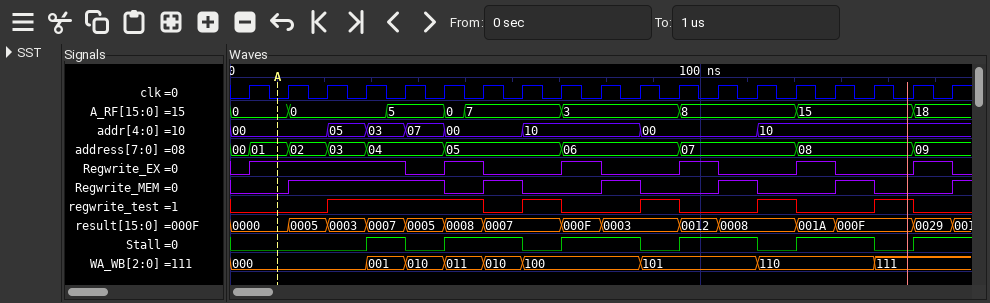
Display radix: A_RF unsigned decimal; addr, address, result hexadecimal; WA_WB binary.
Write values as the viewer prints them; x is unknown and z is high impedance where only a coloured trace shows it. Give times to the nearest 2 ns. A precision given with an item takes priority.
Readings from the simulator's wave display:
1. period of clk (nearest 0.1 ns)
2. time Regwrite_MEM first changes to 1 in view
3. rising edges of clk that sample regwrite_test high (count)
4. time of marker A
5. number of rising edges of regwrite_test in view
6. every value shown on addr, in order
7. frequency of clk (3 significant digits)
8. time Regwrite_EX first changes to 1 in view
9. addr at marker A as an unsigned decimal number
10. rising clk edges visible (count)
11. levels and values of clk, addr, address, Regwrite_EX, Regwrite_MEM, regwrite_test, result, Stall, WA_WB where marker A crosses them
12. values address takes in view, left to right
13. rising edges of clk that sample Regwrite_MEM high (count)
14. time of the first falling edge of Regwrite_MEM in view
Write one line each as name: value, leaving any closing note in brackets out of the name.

period of clk: 8.3 ns
time Regwrite_MEM first changes to 1 in view: 12 ns
rising edges of clk that sample regwrite_test high: 8
time of marker A: 10 ns
number of rising edges of regwrite_test in view: 5
every value shown on addr, in order: 00, 05, 03, 07, 00, 10, 00, 10
frequency of clk: 120 MHz
time Regwrite_EX first changes to 1 in view: 4 ns
addr at marker A as an unsigned decimal number: 0
rising clk edges visible: 19
levels and values of clk, addr, address, Regwrite_EX, Regwrite_MEM, regwrite_test, result, Stall, WA_WB where marker A crosses them: clk=0, addr=00, address=01, Regwrite_EX=1, Regwrite_MEM=0, regwrite_test=0, result=0000, Stall=0, WA_WB=000
values address takes in view, left to right: 00, 01, 02, 03, 04, 05, 06, 07, 08, 09
rising edges of clk that sample Regwrite_MEM high: 8
time of the first falling edge of Regwrite_MEM in view: 46 ns
